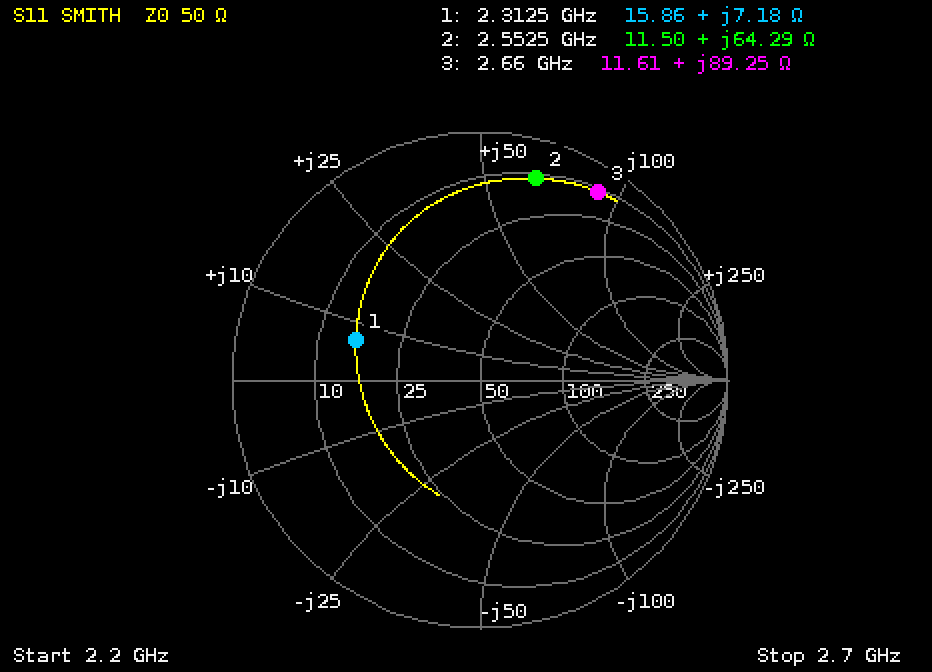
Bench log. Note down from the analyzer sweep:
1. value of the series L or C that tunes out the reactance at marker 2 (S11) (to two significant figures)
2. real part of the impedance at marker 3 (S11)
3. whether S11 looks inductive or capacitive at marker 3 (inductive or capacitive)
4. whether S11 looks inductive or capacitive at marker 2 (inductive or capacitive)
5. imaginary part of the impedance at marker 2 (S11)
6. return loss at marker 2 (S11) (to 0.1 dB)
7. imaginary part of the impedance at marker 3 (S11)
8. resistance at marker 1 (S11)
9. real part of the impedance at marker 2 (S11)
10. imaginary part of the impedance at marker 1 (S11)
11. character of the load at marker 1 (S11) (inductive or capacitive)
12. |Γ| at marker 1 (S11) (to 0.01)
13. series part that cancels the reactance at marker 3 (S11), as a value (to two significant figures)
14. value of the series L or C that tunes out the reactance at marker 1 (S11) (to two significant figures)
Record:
970 fF
11.61 Ω
inductive
inductive
+64.29 Ω
1.5 dB
+89.25 Ω
15.86 Ω
11.50 Ω
+7.18 Ω
inductive
0.53
670 fF
9.6 pF
